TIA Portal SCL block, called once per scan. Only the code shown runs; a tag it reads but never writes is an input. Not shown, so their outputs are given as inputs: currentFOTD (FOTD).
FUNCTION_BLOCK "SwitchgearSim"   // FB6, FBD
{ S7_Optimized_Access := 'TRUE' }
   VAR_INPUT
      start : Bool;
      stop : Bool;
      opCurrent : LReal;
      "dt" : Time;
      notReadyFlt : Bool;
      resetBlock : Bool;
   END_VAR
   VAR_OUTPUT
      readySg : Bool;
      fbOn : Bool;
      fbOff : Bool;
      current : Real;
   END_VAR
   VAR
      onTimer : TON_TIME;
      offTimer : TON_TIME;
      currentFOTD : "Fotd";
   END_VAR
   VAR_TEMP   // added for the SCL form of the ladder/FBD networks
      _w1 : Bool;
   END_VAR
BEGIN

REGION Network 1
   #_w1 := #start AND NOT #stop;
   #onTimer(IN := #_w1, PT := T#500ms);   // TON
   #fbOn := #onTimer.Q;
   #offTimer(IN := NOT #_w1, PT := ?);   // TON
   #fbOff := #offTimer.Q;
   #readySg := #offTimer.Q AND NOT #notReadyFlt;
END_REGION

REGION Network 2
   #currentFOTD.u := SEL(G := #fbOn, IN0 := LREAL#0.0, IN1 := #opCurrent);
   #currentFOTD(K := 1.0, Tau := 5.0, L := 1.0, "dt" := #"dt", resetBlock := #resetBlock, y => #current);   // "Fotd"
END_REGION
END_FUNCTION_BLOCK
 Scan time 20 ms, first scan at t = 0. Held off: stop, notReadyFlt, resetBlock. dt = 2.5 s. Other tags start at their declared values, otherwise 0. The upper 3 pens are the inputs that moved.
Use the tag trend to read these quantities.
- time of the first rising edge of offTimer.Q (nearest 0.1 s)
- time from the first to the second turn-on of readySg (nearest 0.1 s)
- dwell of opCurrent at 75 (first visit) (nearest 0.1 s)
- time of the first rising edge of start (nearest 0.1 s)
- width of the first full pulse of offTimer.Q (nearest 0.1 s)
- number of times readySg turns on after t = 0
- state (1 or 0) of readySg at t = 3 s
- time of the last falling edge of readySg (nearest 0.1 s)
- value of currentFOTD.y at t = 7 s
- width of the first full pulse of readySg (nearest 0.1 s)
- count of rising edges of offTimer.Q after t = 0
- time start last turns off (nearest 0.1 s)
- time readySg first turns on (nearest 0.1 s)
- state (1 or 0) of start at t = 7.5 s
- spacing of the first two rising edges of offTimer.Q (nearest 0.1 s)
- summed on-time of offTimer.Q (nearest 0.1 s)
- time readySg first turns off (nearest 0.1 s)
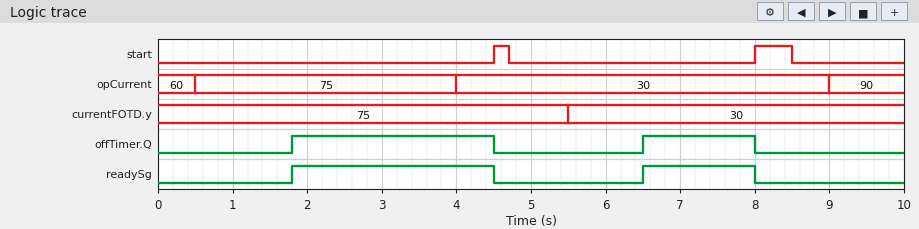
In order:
1.8 s
4.7 s
3.5 s
4.5 s
2.7 s
2
1
8.0 s
30
2.7 s
2
8.5 s
1.8 s
0
4.7 s
4.2 s
4.5 s
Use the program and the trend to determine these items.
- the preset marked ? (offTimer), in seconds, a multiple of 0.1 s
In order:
1.8 s
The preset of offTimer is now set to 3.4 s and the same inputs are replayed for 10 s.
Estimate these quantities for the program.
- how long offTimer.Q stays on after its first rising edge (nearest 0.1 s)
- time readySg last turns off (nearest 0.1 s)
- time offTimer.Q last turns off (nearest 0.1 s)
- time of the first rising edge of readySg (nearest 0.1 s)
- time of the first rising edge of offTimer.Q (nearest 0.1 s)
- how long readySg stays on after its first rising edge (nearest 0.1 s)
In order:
1.1 s
4.5 s
4.5 s
3.4 s
3.4 s
1.1 s
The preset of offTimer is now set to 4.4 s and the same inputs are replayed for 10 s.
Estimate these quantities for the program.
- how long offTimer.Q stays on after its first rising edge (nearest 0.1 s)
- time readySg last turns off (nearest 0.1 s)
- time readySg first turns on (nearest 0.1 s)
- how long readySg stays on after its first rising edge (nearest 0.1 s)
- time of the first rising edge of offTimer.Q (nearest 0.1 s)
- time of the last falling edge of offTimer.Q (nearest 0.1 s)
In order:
0.1 s
4.5 s
4.4 s
0.1 s
4.4 s
4.5 s
